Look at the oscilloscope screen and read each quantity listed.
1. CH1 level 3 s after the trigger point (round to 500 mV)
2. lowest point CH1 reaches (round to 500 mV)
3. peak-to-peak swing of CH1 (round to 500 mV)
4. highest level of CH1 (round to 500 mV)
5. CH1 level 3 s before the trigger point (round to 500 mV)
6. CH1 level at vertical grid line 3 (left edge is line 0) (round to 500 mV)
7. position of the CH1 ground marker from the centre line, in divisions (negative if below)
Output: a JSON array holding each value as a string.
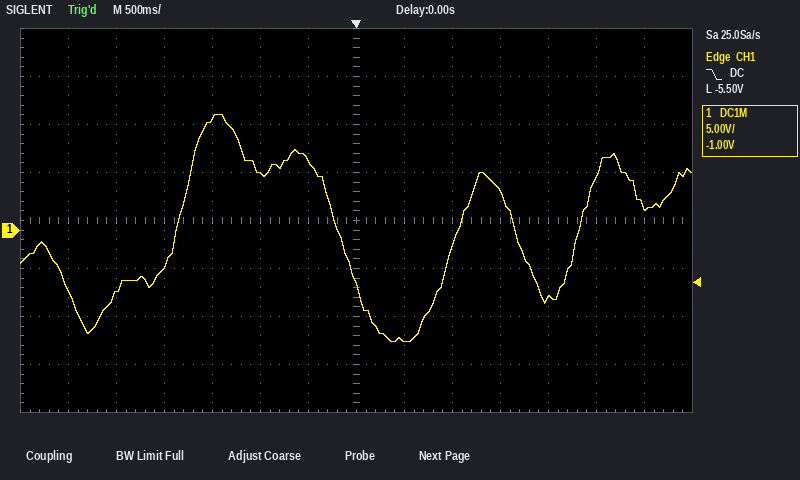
["2.5 V", "-11.5 V", "23.5 V", "12.0 V", "-6.5 V", "-4.0 V", "-0.2 div"]
